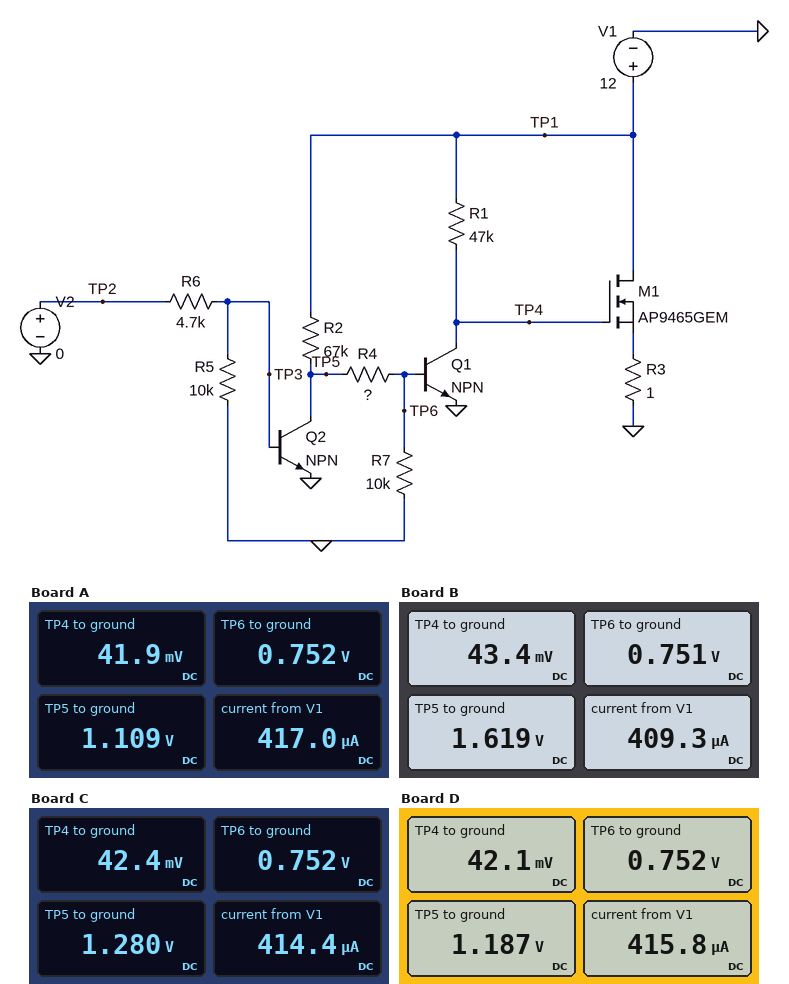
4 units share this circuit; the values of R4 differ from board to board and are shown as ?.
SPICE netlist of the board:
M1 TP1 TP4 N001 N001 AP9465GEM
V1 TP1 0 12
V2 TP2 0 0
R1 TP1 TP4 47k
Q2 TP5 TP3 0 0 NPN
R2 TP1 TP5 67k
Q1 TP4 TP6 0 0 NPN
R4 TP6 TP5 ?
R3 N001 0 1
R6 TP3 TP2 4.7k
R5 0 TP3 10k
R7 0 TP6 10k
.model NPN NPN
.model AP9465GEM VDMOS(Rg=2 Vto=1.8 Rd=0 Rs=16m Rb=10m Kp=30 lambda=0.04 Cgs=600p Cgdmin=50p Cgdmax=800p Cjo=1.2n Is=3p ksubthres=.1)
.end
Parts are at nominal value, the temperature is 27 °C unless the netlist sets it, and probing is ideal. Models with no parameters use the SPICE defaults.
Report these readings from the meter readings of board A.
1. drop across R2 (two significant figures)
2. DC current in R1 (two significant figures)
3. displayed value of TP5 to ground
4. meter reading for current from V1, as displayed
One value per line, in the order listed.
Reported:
11 V
250 µA
1.109 V
417.0 µA
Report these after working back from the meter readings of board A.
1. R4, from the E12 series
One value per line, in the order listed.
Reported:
2.2 kΩ
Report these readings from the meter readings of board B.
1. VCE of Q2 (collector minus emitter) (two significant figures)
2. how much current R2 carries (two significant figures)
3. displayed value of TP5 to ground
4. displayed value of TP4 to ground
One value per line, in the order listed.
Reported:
1.6 V
150 µA
1.619 V
43.4 mV
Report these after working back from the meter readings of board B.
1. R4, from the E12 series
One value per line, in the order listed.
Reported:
5.6 kΩ
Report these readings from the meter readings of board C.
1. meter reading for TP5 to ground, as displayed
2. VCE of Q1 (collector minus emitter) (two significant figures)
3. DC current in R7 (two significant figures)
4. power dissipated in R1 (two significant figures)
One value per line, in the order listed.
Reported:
1.280 V
42 mV
75 µA
3.0 mW
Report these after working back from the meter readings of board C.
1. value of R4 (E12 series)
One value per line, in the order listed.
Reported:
3.3 kΩ
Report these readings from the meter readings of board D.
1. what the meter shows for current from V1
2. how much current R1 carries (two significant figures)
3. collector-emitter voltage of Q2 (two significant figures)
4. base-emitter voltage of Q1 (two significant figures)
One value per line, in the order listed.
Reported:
415.8 µA
250 µA
1.2 V
750 mV
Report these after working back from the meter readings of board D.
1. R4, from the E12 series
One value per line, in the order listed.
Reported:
2.7 kΩ
